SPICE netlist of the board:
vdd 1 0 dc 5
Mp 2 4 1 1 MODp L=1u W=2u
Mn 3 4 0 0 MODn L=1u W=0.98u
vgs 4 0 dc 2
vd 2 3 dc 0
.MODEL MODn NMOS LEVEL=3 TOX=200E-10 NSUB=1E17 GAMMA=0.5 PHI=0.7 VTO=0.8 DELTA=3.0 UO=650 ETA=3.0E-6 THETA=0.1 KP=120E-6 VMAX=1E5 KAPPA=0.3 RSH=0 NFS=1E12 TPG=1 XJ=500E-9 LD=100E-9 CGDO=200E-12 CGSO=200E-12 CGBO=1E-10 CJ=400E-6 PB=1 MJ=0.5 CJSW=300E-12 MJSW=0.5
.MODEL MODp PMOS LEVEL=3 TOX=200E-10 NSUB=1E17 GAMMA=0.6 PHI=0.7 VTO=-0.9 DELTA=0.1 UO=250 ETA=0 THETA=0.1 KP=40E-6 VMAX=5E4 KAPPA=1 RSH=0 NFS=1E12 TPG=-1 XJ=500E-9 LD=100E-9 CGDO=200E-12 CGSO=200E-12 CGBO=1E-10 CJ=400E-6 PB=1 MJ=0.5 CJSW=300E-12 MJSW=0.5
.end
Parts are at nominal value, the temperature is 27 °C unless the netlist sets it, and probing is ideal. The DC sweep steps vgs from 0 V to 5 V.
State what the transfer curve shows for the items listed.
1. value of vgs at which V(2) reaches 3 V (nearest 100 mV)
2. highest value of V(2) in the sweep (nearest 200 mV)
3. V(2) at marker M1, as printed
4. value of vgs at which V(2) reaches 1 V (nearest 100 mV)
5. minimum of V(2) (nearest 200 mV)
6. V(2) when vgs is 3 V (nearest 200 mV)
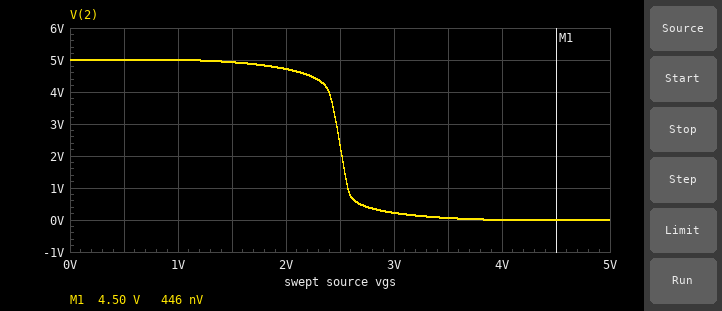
2.5 V
5.0 V
446 nV
2.6 V
0 V
200 mV
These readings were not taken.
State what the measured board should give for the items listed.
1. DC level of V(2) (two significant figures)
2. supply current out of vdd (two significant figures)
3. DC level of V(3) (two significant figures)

4.7 V
40 µA
4.7 V
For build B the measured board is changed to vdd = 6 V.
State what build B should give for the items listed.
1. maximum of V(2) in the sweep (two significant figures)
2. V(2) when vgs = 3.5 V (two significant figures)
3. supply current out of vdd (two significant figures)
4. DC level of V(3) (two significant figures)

6.0 V
370 mV
41 µA
5.8 V
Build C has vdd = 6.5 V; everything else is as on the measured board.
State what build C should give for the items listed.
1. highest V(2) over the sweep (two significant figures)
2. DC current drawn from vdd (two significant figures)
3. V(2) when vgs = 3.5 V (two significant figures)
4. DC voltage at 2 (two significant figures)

6.5 V
42 µA
740 mV
6.3 V
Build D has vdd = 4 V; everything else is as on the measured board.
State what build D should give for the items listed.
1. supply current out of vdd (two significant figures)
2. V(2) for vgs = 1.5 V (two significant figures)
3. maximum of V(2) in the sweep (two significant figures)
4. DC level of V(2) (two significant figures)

38 µA
3.9 V
4.0 V
2.3 V
